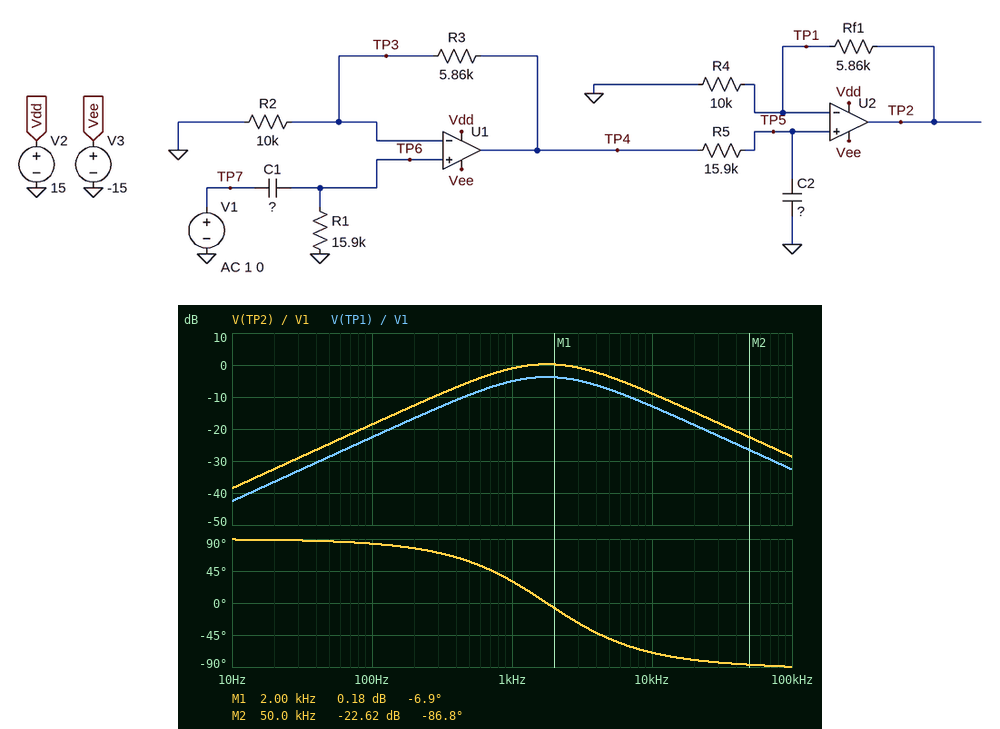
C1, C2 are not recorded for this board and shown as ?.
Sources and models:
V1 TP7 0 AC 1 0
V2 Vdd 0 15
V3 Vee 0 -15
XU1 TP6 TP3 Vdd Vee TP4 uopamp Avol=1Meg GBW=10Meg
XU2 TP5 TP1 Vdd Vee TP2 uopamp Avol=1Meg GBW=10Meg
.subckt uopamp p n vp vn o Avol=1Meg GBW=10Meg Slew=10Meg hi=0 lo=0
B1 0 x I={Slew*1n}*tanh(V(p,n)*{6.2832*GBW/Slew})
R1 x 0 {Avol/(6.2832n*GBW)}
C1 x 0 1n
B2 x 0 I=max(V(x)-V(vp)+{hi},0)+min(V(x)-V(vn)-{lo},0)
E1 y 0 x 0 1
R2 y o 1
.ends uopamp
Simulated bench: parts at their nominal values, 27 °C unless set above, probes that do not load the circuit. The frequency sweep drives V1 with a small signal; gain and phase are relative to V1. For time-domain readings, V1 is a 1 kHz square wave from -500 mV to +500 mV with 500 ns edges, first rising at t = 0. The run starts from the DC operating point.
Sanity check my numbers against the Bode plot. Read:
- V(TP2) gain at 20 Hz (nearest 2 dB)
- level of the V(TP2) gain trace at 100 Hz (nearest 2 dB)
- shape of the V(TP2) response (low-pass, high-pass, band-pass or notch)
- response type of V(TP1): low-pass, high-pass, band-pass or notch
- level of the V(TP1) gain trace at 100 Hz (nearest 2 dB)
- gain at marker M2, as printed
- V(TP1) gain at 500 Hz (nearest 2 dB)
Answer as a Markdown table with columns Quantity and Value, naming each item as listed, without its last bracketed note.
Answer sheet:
| Quantity | Value |
|---|---|
| V(TP2) gain at 20 Hz | -32 dB |
| level of the V(TP2) gain trace at 100 Hz | -18 dB |
| shape of the V(TP2) response | band-pass |
| response type of V(TP1): low-pass, high-pass, band-pass or notch | band-pass |
| level of the V(TP1) gain trace at 100 Hz | -22 dB |
| gain at marker M2, as printed | -22.62 dB |
| V(TP1) gain at 500 Hz | -10 dB |
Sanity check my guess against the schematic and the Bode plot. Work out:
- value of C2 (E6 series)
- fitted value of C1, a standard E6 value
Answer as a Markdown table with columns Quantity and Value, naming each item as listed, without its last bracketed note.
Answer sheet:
| Quantity | Value |
|---|---|
| value of C2 | 6.8 nF |
| fitted value of C1, a standard E6 value | 4.7 nF |
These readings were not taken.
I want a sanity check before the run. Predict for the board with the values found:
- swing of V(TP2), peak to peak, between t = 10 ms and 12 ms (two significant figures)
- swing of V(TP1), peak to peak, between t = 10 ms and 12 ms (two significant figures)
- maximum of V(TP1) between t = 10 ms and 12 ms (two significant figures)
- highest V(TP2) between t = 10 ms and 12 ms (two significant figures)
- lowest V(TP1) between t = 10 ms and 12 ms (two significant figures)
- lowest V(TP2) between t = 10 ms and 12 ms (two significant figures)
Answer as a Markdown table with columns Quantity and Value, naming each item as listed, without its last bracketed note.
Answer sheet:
| Quantity | Value |
|---|---|
| swing of V(TP2), peak to peak, between t = 10 ms and 12 ms | 1.5 V |
| swing of V(TP1), peak to peak, between t = 10 ms and 12 ms | 930 mV |
| maximum of V(TP1) between t = 10 ms and 12 ms | 470 mV |
| highest V(TP2) between t = 10 ms and 12 ms | 740 mV |
| lowest V(TP1) between t = 10 ms and 12 ms | -470 mV |
| lowest V(TP2) between t = 10 ms and 12 ms | -740 mV |
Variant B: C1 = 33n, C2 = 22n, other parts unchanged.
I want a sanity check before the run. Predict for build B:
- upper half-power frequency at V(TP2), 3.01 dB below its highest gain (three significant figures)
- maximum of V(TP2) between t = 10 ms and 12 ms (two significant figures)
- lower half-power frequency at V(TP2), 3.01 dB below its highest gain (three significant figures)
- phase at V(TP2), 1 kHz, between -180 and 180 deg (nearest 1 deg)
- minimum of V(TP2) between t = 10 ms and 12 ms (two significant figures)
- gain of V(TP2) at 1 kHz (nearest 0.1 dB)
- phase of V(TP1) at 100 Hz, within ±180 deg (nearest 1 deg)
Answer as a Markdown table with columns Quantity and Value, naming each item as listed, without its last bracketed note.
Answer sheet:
| Quantity | Value |
|---|---|
| upper half-power frequency at V(TP2), 3.01 dB below its highest gain | 910 Hz |
| maximum of V(TP2) between t = 10 ms and 12 ms | 640 mV |
| lower half-power frequency at V(TP2), 3.01 dB below its highest gain | 152 Hz |
| phase at V(TP2), 1 kHz, between -180 and 180 deg | -49 deg |
| minimum of V(TP2) between t = 10 ms and 12 ms | -640 mV |
| gain of V(TP2) at 1 kHz | 0 dB |
| phase of V(TP1) at 100 Hz, within ±180 deg | 59 deg |
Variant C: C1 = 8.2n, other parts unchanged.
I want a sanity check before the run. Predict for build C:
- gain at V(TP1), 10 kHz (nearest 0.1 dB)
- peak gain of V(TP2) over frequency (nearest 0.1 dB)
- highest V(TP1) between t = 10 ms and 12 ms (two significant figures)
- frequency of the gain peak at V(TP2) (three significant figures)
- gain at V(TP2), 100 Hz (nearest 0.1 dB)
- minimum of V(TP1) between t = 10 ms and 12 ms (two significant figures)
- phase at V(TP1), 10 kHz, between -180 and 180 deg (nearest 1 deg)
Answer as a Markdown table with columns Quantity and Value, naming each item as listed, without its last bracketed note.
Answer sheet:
| Quantity | Value |
|---|---|
| gain at V(TP1), 10 kHz | -12.8 dB |
| peak gain of V(TP2) over frequency | 2.8 dB |
| highest V(TP1) between t = 10 ms and 12 ms | 590 mV |
| frequency of the gain peak at V(TP2) | 1.34 kHz |
| gain at V(TP2), 100 Hz | -13.8 dB |
| minimum of V(TP1) between t = 10 ms and 12 ms | -590 mV |
| phase at V(TP1), 10 kHz, between -180 and 180 deg | -75 deg |
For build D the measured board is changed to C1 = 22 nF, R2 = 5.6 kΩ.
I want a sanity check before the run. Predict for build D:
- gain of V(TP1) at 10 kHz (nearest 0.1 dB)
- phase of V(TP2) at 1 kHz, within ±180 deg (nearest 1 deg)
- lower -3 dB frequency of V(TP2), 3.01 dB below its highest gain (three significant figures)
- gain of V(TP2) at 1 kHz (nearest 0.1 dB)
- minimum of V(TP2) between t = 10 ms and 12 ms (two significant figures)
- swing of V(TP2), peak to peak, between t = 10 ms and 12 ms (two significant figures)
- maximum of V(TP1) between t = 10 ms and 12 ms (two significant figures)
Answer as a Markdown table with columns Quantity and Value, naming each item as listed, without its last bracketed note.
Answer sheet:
| Quantity | Value |
|---|---|
| gain of V(TP1) at 10 kHz | -10.5 dB |
| phase of V(TP2) at 1 kHz, within ±180 deg | -10 deg |
| lower -3 dB frequency of V(TP2), 3.01 dB below its highest gain | 301 Hz |
| gain of V(TP2) at 1 kHz | 7.8 dB |
| minimum of V(TP2) between t = 10 ms and 12 ms | -1.4 V |
| swing of V(TP2), peak to peak, between t = 10 ms and 12 ms | 2.8 V |
| maximum of V(TP1) between t = 10 ms and 12 ms | 890 mV |
